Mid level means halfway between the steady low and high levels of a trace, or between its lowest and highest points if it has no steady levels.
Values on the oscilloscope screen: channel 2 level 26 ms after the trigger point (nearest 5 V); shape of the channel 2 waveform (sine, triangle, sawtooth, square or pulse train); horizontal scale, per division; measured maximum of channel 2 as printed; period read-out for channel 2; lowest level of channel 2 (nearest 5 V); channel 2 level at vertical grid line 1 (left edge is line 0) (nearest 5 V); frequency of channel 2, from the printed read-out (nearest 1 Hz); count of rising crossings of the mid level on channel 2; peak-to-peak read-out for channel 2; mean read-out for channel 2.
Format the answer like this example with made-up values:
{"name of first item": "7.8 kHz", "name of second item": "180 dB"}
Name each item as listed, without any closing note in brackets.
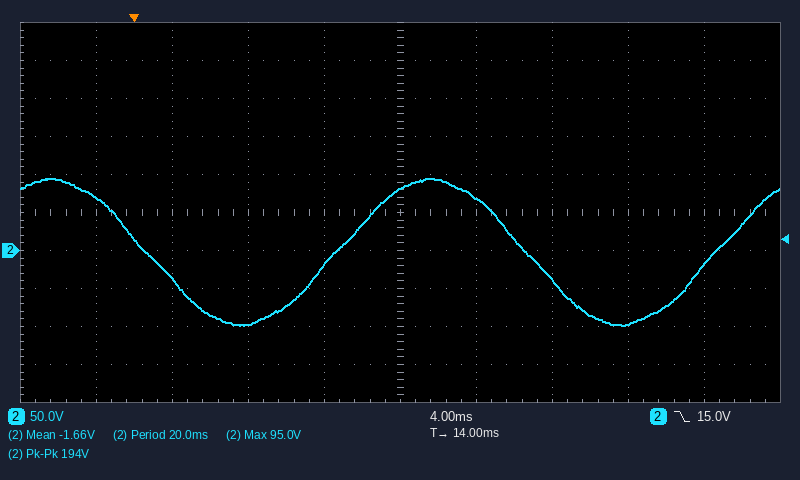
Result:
{"channel 2 level 26 ms after the trigger point": "-95 V", "shape of the channel 2 waveform": "sine", "horizontal scale, per division": "4 ms", "measured maximum of channel 2 as printed": "95.0 V", "period read-out for channel 2": "20.0 ms", "lowest level of channel 2": "-100 V", "channel 2 level at vertical grid line 1 (left edge is line 0)": "70 V", "frequency of channel 2, from the printed read-out": "50 Hz", "count of rising crossings of the mid level on channel 2": "2", "peak-to-peak read-out for channel 2": "194 V", "mean read-out for channel 2": "-1.66 V"}
